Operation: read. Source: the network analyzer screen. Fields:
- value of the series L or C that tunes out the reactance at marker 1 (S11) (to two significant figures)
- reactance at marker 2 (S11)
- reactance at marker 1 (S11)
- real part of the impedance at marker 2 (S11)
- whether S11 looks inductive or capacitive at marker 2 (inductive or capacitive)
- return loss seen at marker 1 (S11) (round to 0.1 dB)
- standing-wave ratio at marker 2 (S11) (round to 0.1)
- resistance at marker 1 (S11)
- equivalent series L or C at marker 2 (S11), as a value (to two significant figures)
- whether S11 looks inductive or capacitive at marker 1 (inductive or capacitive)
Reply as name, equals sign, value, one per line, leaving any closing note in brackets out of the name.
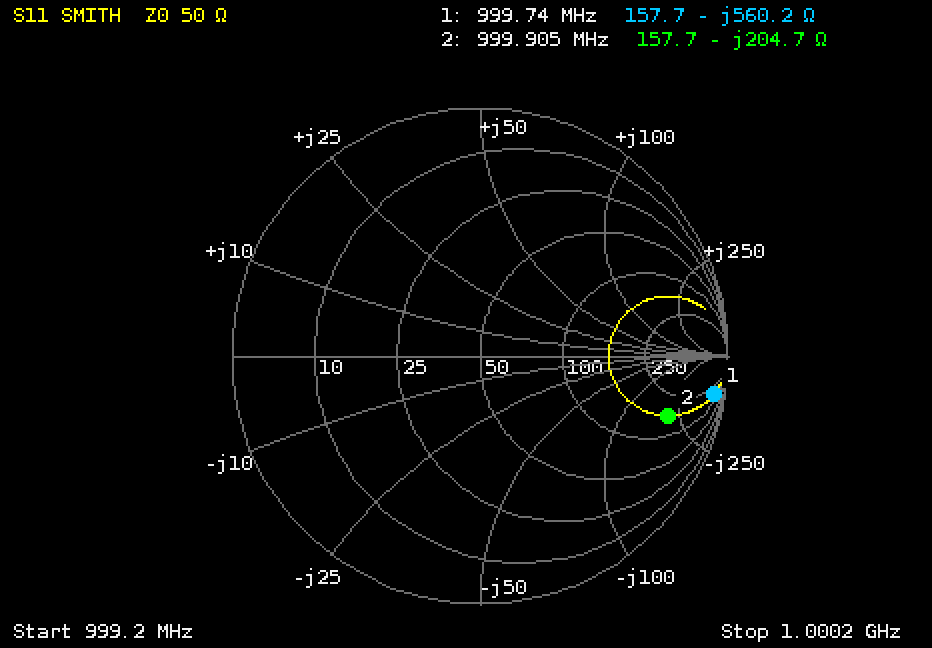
value of the series L or C that tunes out the reactance at marker 1 (S11) = 89 nH
reactance at marker 2 = -204.7 Ω
reactance at marker 1 = -560.2 Ω
real part of the impedance at marker 2 = 157.7 Ω
whether S11 looks inductive or capacitive at marker 2 = capacitive
return loss seen at marker 1 (S11) = 0.4 dB
standing-wave ratio at marker 2 (S11) = 8.7
resistance at marker 1 = 157.7 Ω
equivalent series L or C at marker 2 (S11), as a value = 780 fF
whether S11 looks inductive or capacitive at marker 1 = capacitive
